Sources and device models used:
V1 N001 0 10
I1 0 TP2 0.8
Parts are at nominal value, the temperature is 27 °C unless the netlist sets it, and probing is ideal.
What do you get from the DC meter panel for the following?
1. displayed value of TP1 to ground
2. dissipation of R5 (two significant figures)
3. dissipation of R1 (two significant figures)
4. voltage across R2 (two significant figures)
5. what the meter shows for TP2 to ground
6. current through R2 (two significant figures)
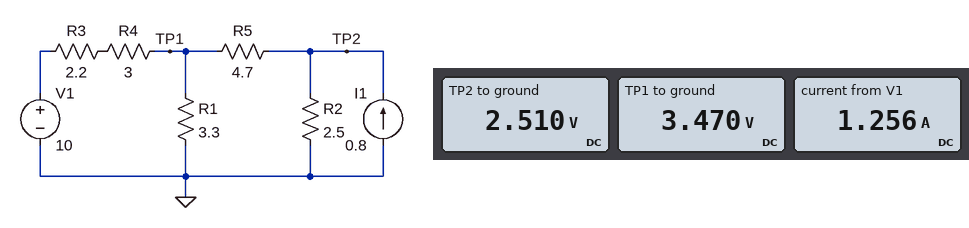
3.470 V
200 mW
3.6 W
2.5 V
2.510 V
1.0 A
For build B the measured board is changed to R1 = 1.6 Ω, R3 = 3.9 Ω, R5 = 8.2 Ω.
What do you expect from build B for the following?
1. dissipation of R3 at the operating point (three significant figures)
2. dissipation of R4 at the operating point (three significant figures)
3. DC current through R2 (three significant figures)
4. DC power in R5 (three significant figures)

5.38 W
4.14 W
790 mA
788 µW
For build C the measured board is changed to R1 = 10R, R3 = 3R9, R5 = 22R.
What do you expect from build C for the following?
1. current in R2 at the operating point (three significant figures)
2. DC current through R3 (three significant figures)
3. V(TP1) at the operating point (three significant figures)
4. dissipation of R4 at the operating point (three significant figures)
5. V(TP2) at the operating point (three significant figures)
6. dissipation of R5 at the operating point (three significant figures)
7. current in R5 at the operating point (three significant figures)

937 mA
673 mA
5.36 V
1.36 W
2.34 V
413 mW
137 mA
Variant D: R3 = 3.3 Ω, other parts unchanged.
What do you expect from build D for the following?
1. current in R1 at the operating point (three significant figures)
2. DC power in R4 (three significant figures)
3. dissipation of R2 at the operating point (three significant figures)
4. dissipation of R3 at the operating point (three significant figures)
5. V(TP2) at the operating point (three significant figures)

941 mA
3.59 W
2.27 W
3.95 W
2.38 V
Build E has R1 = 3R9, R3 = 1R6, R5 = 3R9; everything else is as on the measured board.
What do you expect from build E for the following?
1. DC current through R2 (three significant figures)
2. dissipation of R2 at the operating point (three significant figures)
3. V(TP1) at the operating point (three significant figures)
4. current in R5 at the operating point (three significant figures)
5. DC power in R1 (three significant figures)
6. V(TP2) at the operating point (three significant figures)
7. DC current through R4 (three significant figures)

1.10 A
3.05 W
3.95 V
304 mA
3.99 W
2.76 V
1.32 A
